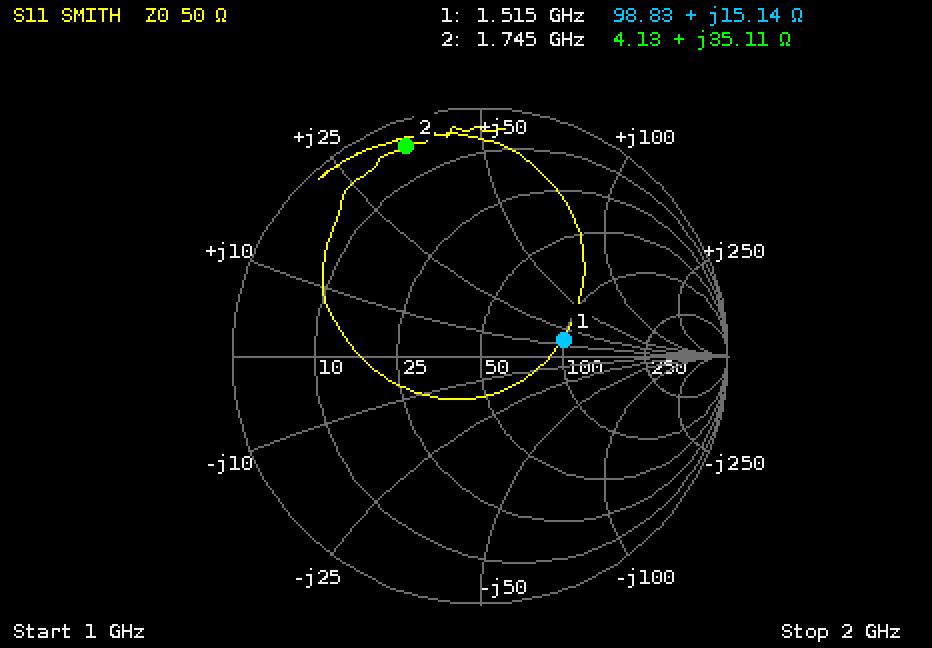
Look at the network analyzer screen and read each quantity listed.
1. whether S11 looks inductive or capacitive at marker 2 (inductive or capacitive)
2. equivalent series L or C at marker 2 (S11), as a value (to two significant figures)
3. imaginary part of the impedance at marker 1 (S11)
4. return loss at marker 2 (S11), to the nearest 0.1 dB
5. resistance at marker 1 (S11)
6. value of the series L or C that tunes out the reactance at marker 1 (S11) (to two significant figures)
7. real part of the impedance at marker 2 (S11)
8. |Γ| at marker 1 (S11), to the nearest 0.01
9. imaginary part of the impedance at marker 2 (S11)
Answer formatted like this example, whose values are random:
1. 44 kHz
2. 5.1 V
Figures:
1. inductive
2. 3.2 nH
3. +15.14 Ω
4. 1.0 dB
5. 98.83 Ω
6. 6.9 pF
7. 4.13 Ω
8. 0.34
9. +35.11 Ω
